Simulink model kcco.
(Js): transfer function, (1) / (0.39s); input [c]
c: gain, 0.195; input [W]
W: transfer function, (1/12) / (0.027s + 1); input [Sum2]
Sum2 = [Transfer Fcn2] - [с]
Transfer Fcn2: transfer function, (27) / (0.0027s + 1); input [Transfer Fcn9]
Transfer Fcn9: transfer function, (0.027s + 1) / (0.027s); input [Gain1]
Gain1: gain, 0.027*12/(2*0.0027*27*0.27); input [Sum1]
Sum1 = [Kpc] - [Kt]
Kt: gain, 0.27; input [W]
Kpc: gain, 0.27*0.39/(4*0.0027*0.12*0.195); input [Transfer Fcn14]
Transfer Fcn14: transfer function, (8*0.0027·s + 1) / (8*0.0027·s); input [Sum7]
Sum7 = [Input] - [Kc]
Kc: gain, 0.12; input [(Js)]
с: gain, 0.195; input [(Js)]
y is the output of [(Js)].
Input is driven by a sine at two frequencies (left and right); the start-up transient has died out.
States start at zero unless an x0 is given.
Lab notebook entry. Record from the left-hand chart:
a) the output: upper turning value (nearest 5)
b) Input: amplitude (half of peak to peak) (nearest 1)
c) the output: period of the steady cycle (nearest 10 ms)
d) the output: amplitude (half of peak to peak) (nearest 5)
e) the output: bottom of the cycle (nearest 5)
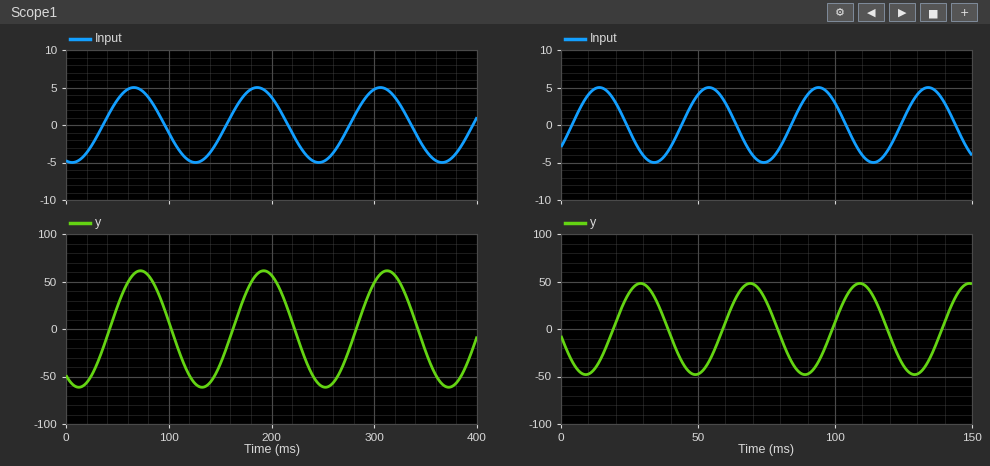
60
5
120 ms
60
-60
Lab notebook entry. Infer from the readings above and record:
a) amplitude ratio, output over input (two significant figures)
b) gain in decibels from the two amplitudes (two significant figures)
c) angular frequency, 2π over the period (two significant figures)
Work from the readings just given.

12
22 dB
0.052 rad/ms
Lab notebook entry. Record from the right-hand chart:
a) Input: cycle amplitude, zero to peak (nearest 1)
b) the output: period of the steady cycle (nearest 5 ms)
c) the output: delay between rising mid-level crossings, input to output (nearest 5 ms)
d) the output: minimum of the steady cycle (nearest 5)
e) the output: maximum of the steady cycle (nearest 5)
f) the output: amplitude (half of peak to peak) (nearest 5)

5
40 ms
15 ms
-50
50
50
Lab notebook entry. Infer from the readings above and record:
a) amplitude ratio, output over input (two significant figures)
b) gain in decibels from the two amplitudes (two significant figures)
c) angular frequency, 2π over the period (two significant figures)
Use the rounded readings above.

10
20 dB
0.16 rad/ms
